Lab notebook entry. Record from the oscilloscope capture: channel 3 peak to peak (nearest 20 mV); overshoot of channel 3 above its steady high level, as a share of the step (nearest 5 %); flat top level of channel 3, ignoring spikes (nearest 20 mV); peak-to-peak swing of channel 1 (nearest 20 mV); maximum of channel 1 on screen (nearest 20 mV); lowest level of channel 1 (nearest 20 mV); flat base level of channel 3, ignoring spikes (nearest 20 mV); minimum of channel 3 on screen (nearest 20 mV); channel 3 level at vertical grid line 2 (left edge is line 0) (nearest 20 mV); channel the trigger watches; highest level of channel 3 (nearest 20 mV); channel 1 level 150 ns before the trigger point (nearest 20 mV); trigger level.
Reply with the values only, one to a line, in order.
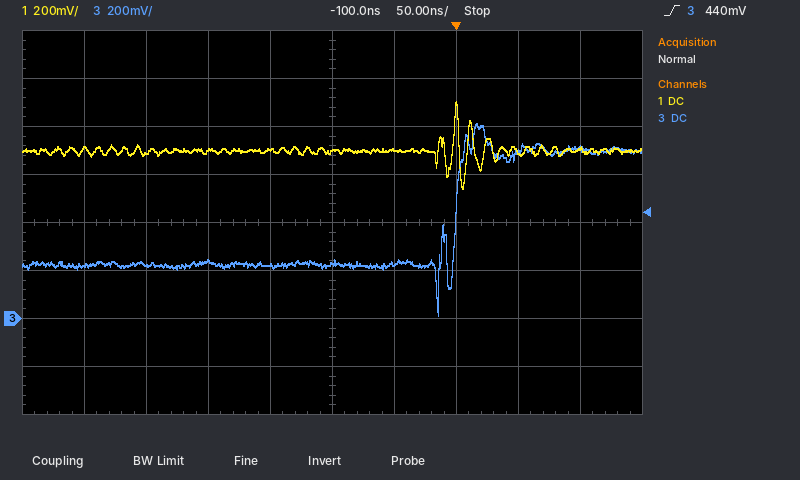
800 mV
25 %
700 mV
360 mV
900 mV
540 mV
220 mV
20 mV
220 mV
channel 3
820 mV
700 mV
440 mV
